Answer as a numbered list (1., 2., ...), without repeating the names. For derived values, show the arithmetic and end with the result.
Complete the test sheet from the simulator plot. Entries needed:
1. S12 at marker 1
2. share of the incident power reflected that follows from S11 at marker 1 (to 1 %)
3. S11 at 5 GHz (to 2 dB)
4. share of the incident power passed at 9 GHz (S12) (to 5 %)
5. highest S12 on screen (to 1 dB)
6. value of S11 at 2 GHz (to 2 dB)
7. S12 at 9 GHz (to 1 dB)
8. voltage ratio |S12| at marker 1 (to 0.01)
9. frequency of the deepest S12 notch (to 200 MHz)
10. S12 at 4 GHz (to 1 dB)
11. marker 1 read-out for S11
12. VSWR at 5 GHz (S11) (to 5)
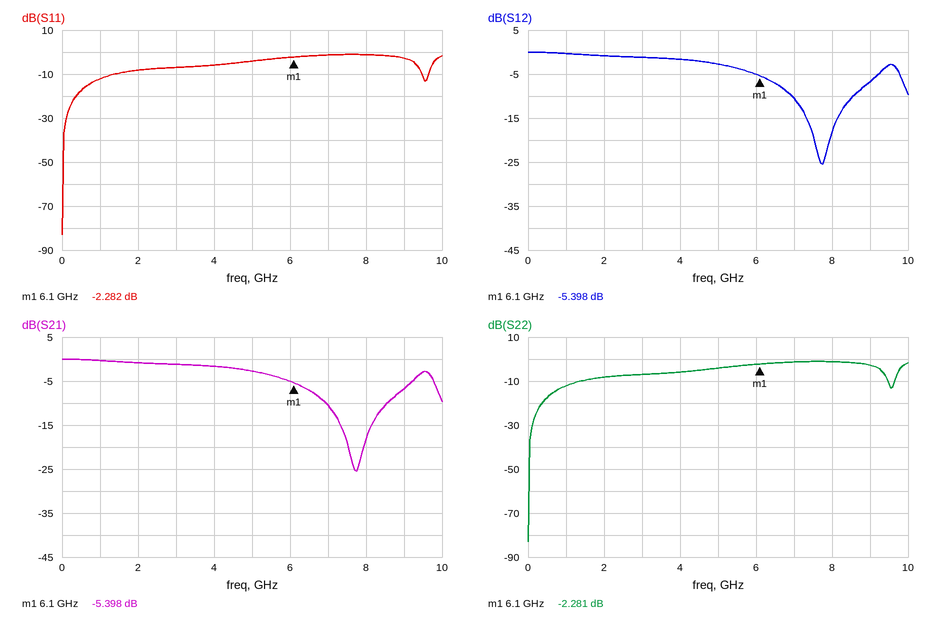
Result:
1. -5.398 dB
2. 10^(-2.282/10) ≈ 59 %
3. -4 dB
4. 10^(-7/10) ≈ 20 %
5. 0 dB
6. -8 dB
7. -7 dB
8. 10^(-5.398/20) ≈ 0.54
9. 7.8 GHz
10. -2 dB
11. -2.282 dB
12. |Γ| = 10^(-4/20) = 0.6310; VSWR = (1 + 0.6310)/(1 − 0.6310) ≈ 4.42, so 5 to the nearest 5
